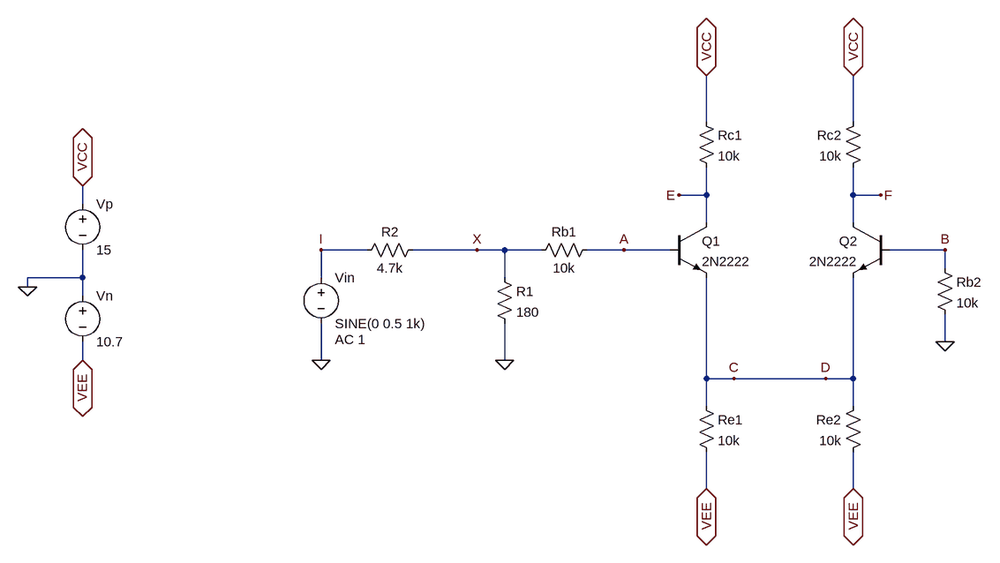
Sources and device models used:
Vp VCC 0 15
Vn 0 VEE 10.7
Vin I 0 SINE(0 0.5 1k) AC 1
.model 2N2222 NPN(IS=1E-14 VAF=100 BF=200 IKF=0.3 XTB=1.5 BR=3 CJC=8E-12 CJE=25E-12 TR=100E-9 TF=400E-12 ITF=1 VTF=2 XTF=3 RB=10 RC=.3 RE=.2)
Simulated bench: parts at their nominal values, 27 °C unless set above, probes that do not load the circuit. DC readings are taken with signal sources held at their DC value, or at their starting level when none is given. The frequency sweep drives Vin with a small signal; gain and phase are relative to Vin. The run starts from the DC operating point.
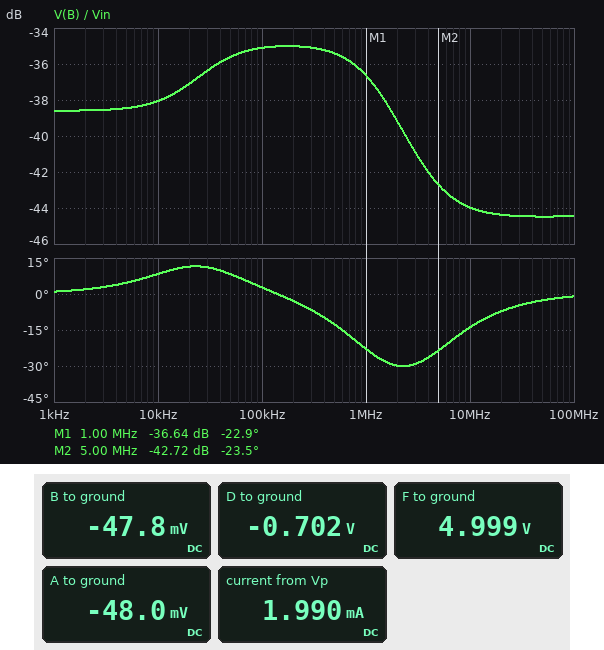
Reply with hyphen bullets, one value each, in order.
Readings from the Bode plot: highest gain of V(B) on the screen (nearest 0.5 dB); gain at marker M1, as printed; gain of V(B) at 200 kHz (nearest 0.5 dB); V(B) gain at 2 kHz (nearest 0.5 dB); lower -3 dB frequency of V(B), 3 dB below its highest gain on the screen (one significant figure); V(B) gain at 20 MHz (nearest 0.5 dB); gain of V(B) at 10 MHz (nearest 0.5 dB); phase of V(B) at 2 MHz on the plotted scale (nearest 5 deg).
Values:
- -35.0 dB
- -36.64 dB
- -35.0 dB
- -38.5 dB
- 10 kHz
- -44.5 dB
- -44.0 dB
- -30 deg
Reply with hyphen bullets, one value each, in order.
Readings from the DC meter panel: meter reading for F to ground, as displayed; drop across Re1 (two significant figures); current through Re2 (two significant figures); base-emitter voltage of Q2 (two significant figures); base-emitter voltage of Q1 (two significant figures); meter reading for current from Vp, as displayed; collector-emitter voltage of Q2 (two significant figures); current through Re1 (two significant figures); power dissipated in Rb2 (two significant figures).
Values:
- 4.999 V
- 10 V
- 1.0 mA
- 650 mV
- 650 mV
- 1.990 mA
- 5.7 V
- 1.0 mA
- 230 nW
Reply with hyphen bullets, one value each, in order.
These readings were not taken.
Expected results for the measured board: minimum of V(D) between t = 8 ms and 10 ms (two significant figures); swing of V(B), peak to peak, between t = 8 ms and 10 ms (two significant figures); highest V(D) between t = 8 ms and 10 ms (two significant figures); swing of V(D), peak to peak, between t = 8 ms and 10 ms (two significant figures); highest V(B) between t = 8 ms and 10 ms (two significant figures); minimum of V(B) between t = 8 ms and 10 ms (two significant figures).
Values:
- -710 mV
- 12 mV
- -690 mV
- 18 mV
- -42 mV
- -54 mV
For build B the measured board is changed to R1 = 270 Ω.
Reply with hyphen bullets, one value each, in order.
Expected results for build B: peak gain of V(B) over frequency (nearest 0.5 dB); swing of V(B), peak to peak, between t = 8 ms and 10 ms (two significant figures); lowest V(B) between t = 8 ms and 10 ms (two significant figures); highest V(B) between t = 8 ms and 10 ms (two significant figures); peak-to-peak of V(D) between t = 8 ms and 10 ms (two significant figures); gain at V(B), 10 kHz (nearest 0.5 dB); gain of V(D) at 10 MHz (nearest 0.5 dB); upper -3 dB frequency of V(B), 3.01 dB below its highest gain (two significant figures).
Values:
- -31.5 dB
- 17 mV
- -57 mV
- -39 mV
- 27 mV
- -34.5 dB
- -40.5 dB
- 1.5 MHz
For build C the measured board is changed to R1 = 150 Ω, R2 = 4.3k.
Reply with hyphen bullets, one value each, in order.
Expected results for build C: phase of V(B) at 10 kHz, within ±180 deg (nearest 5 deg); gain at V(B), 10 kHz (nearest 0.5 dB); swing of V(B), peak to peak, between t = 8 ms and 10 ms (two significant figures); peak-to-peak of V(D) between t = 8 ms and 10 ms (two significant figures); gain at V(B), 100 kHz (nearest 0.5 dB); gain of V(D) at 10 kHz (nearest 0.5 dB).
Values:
- 10 deg
- -39.0 dB
- 11 mV
- 17 mV
- -36.0 dB
- -35.5 dB
